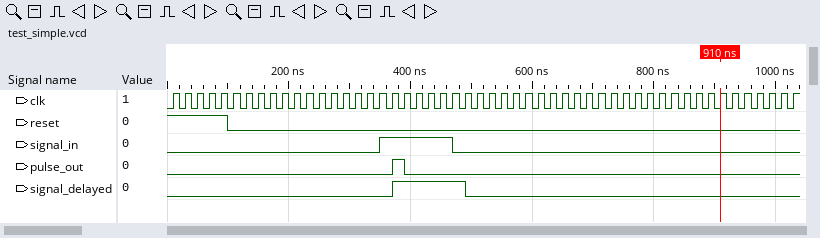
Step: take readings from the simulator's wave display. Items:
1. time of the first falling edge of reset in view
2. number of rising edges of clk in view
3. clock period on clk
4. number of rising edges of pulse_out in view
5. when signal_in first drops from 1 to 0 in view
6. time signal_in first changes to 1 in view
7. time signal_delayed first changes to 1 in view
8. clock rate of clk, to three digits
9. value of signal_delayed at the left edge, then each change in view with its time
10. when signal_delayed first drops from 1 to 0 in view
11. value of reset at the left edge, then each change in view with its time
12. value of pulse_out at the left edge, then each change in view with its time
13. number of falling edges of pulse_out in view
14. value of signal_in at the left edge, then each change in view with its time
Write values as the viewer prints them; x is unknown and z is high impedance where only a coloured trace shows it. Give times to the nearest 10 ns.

100 ns
52
20 ns
1
470 ns
350 ns
370 ns
50.0 MHz
0, 1 at 370 ns, 0 at 490 ns
490 ns
1, 0 at 100 ns
0, 1 at 370 ns, 0 at 390 ns
1
0, 1 at 350 ns, 0 at 470 ns
